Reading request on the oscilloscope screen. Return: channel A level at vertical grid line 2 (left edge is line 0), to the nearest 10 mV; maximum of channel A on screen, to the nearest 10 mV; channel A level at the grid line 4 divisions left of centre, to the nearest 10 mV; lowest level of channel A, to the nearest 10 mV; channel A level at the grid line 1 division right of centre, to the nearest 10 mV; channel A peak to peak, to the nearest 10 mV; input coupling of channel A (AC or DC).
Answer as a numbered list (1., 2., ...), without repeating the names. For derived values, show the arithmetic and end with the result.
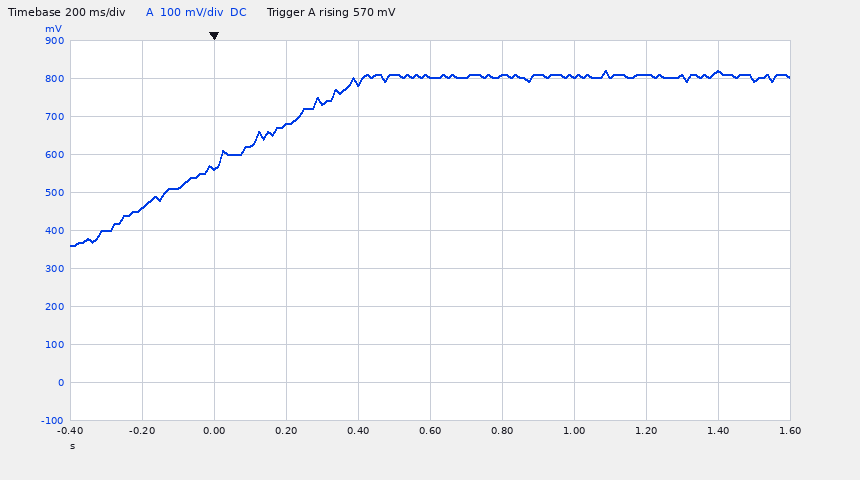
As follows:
1. 560 mV
2. 820 mV
3. 460 mV
4. 360 mV
5. 810 mV
6. 820 mV − (360 mV) = 460 mV
7. DC
